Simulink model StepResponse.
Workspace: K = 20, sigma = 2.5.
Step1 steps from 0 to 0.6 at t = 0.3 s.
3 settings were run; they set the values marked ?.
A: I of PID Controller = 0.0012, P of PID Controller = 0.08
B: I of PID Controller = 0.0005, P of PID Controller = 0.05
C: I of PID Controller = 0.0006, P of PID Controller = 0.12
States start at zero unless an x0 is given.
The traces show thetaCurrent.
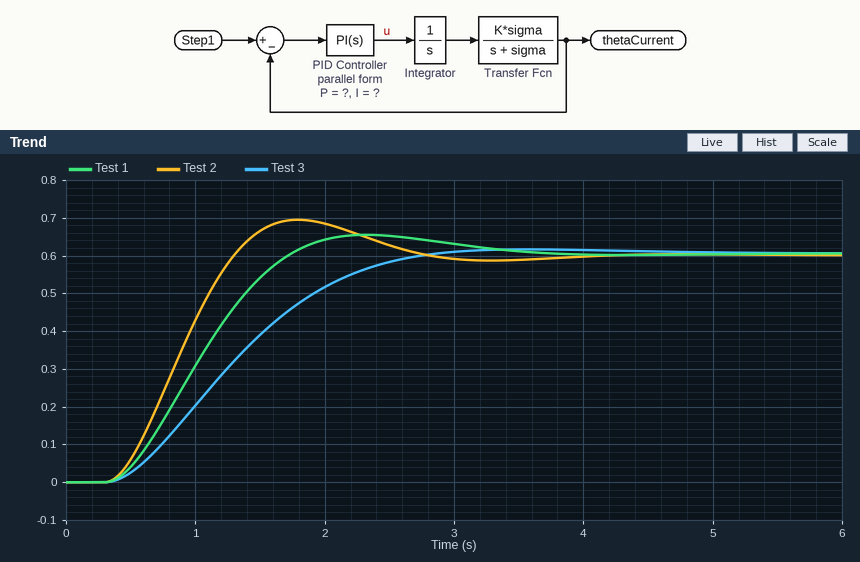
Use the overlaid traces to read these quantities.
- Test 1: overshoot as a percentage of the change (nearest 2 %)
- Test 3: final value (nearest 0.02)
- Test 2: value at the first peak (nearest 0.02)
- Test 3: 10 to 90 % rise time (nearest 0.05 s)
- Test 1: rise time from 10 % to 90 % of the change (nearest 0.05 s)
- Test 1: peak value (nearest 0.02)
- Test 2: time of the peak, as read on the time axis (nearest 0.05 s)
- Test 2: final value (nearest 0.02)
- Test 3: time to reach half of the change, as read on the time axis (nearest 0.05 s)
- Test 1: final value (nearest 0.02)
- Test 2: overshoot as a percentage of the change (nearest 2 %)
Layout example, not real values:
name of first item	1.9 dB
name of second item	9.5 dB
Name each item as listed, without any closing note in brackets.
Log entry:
Test 1: overshoot as a percentage of the change	8 %
Test 3: final value	0.60
Test 2: value at the first peak	0.70
Test 3: 10 to 90 % rise time	1.55 s
Test 1: rise time from 10 % to 90 % of the change	0.95 s
Test 1: peak value	0.66
Test 2: time of the peak, as read on the time axis	1.80 s
Test 2: final value	0.60
Test 3: time to reach half of the change, as read on the time axis	1.25 s
Test 1: final value	0.60
Test 2: overshoot as a percentage of the change	16 %
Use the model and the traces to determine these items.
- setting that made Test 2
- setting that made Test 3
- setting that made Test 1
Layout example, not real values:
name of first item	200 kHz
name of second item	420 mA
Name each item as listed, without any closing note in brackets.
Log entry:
setting that made Test 2	C
setting that made Test 3	B
setting that made Test 1	A
